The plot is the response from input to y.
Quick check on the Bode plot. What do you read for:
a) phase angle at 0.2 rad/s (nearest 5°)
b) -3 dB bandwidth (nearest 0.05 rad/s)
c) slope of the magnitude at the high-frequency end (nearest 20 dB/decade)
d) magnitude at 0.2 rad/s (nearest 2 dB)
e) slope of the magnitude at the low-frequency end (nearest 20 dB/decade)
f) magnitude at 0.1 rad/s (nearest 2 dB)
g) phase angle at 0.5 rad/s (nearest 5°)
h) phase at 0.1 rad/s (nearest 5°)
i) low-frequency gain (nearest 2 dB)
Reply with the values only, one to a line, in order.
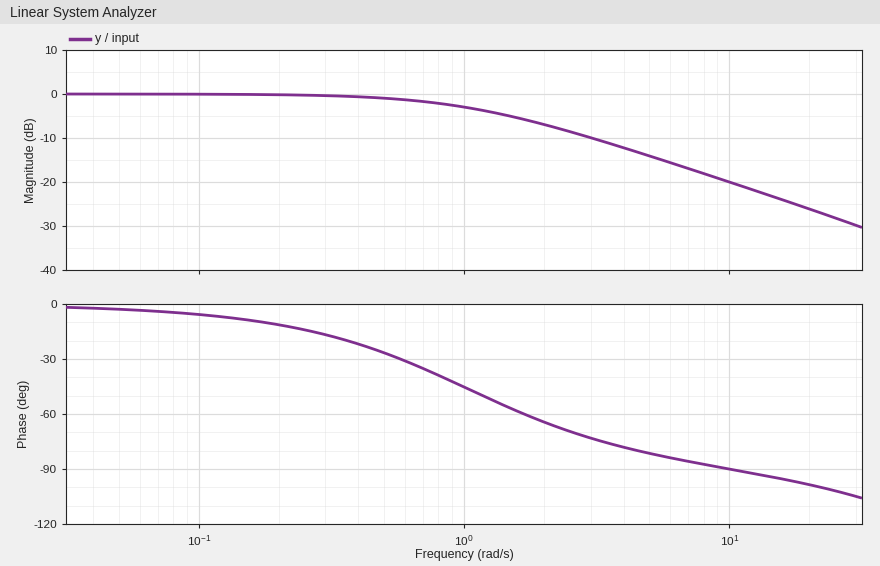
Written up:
-10°
1.00 rad/s
-20 dB/decade
0 dB
0 dB/decade
0 dB
-25°
-5°
0 dB
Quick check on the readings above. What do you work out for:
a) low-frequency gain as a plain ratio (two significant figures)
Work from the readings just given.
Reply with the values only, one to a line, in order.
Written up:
1.0
